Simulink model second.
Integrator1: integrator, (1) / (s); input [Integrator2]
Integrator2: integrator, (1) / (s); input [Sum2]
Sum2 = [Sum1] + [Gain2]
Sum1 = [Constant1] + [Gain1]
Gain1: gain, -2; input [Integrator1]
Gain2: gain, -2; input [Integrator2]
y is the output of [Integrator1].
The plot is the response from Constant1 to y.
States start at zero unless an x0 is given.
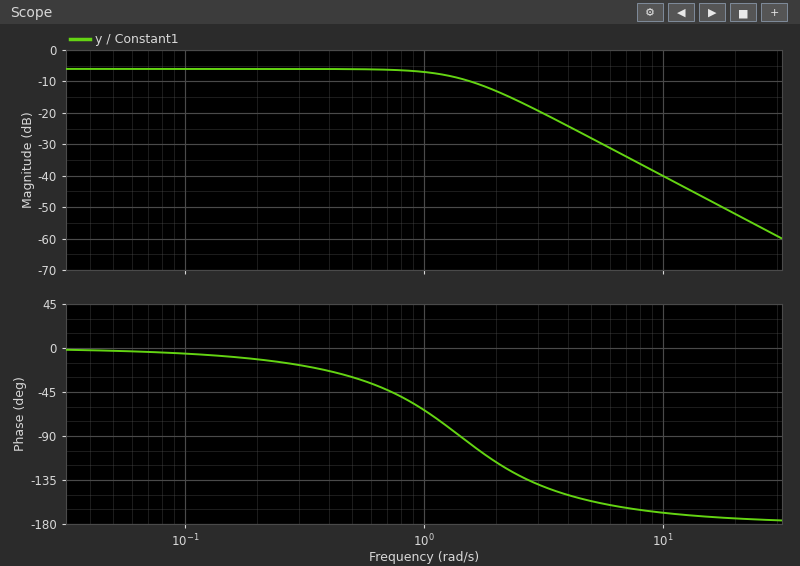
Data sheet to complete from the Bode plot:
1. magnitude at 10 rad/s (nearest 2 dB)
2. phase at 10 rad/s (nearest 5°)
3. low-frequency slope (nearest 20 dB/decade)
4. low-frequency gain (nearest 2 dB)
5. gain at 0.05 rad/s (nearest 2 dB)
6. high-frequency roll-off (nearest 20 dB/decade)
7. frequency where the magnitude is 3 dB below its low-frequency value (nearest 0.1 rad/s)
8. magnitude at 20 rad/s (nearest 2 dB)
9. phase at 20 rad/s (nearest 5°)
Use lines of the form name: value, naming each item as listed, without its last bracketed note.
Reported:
magnitude at 10 rad/s: -40 dB
phase at 10 rad/s: -170°
low-frequency slope: 0 dB/decade
low-frequency gain: -6 dB
gain at 0.05 rad/s: -6 dB
high-frequency roll-off: -40 dB/decade
frequency where the magnitude is 3 dB below its low-frequency value: 1.4 rad/s
magnitude at 20 rad/s: -52 dB
phase at 20 rad/s: -175°
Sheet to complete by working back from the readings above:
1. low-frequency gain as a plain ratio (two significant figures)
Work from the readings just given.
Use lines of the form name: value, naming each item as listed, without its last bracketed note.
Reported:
low-frequency gain as a plain ratio: 0.50
